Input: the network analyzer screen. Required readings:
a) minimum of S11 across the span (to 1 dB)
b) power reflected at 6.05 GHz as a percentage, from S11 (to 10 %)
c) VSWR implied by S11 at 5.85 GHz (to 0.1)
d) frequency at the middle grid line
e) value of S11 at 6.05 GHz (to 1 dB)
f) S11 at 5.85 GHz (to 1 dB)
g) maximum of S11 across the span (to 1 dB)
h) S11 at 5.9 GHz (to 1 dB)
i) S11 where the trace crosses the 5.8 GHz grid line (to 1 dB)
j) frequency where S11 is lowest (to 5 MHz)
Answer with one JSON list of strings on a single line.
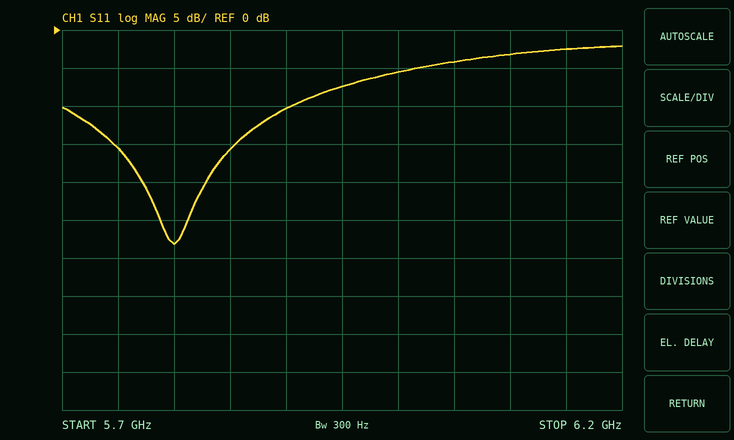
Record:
["-28 dB", "40 %", "1.4", "5.95 GHz", "-4 dB", "-16 dB", "-2 dB", "-10 dB", "-28 dB", "5.800 GHz"]
